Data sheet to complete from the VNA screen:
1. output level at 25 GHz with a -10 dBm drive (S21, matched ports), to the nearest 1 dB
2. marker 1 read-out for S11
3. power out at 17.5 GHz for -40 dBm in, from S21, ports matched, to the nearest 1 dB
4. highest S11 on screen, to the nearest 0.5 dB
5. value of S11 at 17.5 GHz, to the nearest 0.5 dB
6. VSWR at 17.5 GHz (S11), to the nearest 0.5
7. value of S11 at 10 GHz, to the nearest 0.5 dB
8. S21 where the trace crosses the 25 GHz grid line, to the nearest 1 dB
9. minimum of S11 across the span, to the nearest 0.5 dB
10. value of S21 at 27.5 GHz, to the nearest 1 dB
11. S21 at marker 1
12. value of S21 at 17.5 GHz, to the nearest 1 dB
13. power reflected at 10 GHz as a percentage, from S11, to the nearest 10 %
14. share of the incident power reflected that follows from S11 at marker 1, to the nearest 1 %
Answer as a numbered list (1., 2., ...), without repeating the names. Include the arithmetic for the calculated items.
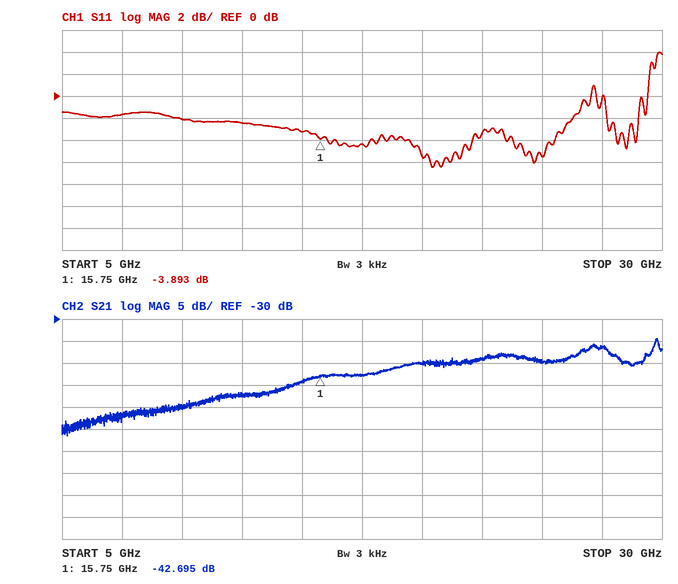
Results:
1. -10 dBm + (-40 dB) = -50 dBm
2. -3.893 dB
3. -40 dBm + (-43 dB) = -83 dBm
4. 4.0 dB
5. -4.5 dB
6. |Γ| = 10^(-4.5/20) = 0.5957; VSWR = (1 + 0.5957)/(1 − 0.5957) ≈ 4.0
7. -2.0 dB
8. -40 dB
9. -6.5 dB
10. -36 dB
11. -42.695 dB
12. -43 dB
13. 10^(-2/10) ≈ 63.1 %, so 60 % to the nearest 10 %
14. 10^(-3.893/10) ≈ 41 %
